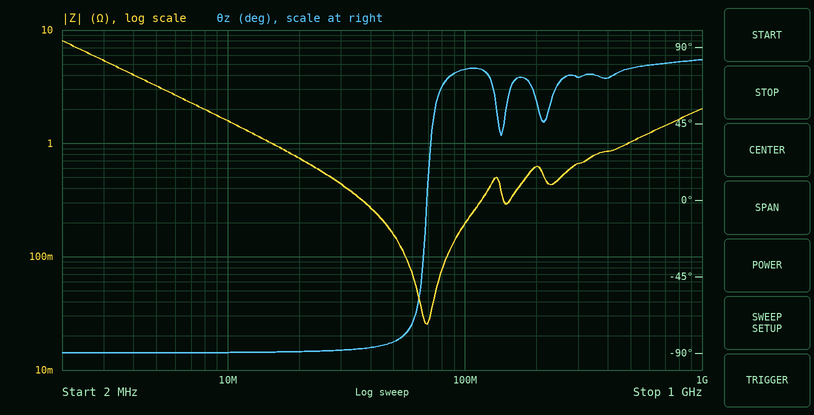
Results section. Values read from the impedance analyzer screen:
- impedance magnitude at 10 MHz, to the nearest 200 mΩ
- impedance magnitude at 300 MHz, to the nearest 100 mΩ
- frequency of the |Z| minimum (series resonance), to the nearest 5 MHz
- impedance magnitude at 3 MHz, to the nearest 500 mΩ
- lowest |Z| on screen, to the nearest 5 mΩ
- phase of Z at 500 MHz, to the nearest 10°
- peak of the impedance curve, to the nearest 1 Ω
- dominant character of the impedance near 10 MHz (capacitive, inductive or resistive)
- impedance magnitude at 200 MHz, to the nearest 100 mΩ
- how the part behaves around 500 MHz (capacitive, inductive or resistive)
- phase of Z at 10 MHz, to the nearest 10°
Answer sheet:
1.6 Ω
700 mΩ
70 MHz
5.5 Ω
25 mΩ
80°
8 Ω
capacitive
600 mΩ
inductive
-90°
